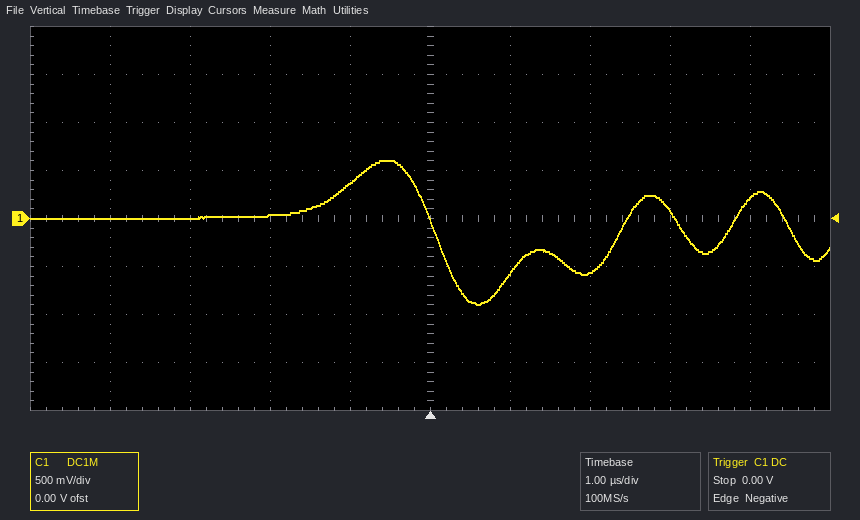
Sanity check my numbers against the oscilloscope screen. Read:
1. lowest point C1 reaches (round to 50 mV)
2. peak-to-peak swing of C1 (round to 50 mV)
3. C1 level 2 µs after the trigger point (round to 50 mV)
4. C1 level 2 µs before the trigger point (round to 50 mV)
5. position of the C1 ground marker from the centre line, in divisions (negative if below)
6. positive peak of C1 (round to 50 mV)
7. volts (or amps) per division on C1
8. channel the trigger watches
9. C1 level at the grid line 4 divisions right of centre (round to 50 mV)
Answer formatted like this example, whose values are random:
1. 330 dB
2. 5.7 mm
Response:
1. -900 mV
2. 1.50 V
3. -550 mV
4. 50 mV
5. 0.0 div
6. 600 mV
7. 500 mV
8. C1
9. 200 mV
